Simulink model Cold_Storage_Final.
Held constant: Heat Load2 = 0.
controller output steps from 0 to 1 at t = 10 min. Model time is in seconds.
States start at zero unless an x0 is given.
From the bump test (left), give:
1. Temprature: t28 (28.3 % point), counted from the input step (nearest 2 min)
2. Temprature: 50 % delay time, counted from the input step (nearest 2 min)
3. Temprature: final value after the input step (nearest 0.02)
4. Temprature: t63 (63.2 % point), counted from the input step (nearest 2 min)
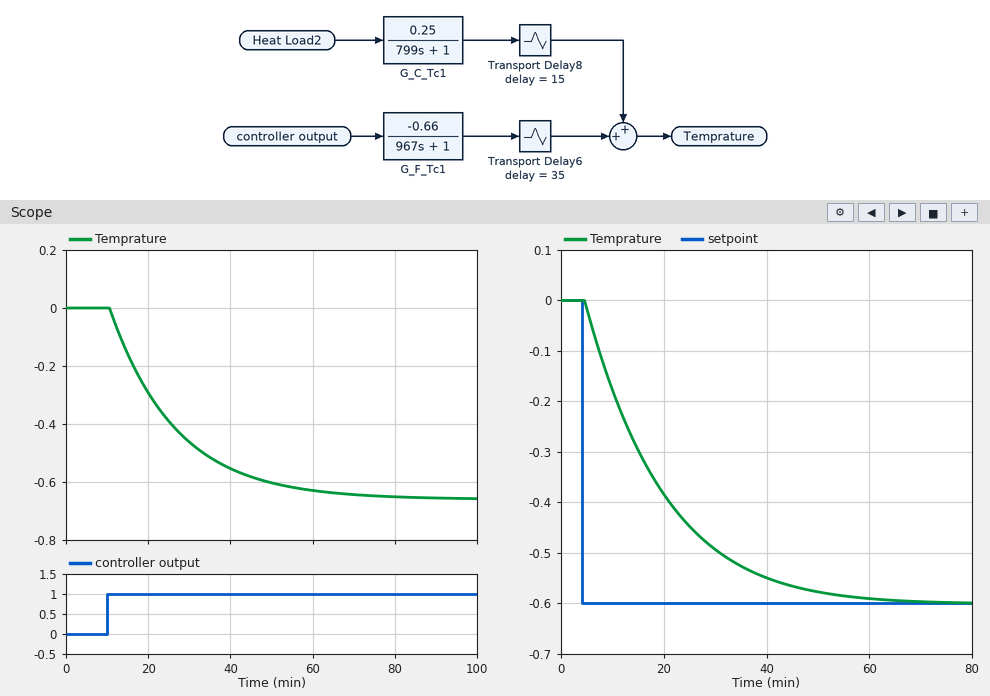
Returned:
6 min
12 min
-0.66
16 min
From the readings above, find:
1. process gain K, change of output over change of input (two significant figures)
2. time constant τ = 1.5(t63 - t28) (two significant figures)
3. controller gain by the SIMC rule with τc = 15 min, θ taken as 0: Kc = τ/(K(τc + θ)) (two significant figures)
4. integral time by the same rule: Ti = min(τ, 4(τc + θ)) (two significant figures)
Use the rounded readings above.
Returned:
-0.66
15 min
-1.5
15 min
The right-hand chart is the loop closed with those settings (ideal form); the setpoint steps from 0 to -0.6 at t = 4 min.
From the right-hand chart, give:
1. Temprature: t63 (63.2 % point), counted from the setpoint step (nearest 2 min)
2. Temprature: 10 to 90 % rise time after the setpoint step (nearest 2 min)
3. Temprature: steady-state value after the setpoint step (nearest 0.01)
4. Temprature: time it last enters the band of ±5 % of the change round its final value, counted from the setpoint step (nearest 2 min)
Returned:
16 min
32 min
-0.60
42 min
